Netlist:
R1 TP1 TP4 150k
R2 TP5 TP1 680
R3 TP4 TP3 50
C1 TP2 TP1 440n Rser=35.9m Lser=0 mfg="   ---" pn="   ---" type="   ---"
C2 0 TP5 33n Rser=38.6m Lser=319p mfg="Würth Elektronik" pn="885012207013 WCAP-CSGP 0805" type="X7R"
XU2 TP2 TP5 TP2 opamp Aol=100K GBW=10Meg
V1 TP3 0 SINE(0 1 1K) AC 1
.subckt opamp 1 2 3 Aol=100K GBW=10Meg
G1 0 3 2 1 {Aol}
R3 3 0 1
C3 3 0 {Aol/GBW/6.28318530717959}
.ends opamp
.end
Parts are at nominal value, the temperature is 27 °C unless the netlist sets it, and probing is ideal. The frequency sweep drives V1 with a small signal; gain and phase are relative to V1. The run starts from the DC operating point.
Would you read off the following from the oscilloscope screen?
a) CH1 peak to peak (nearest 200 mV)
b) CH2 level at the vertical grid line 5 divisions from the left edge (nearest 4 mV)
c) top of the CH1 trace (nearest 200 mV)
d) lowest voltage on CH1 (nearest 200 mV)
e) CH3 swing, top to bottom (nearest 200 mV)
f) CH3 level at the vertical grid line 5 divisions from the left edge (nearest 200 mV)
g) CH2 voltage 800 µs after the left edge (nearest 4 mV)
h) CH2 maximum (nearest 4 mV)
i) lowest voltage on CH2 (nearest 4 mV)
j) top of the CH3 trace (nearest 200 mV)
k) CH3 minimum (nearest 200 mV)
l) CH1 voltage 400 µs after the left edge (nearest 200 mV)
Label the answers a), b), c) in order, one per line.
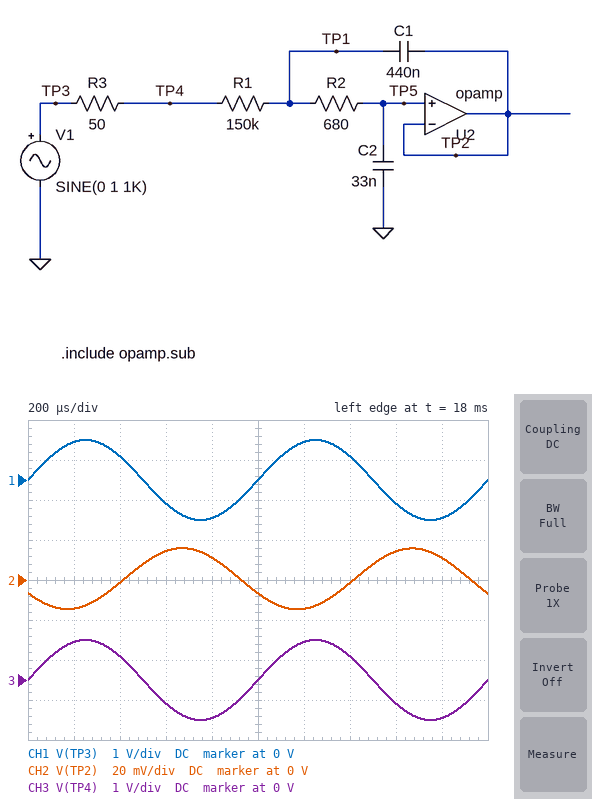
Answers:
a) 2.0 V
b) -8 mV
c) 1.0 V
d) -1.0 V
e) 2.0 V
f) 0 V
g) 12 mV
h) 16 mV
i) -16 mV
j) 1.0 V
k) -1.0 V
l) 600 mV
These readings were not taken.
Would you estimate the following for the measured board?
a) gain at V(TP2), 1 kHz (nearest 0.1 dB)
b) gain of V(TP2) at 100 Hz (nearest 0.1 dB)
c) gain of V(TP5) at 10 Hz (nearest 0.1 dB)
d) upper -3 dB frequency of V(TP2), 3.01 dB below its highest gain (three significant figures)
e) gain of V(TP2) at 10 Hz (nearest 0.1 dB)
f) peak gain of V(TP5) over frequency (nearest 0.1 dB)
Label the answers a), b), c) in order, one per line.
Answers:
a) -36.3 dB
b) -10.0 dB
c) -0.4 dB
d) 34.0 Hz
e) -0.4 dB
f) 0 dB
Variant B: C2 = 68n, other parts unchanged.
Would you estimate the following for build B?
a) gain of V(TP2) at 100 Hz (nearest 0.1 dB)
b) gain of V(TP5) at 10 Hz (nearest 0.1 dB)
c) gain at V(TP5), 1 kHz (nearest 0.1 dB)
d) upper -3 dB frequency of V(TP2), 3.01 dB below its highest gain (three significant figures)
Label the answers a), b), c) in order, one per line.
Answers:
a) -16.2 dB
b) -1.4 dB
c) -42.7 dB
d) 16.0 Hz
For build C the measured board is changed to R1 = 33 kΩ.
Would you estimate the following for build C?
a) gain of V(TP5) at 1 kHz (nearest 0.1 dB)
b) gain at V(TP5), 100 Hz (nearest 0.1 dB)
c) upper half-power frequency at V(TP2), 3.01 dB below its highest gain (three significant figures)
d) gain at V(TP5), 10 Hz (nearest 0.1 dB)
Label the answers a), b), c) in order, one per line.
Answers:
a) -22.8 dB
b) -1.0 dB
c) 186 Hz
d) 0 dB
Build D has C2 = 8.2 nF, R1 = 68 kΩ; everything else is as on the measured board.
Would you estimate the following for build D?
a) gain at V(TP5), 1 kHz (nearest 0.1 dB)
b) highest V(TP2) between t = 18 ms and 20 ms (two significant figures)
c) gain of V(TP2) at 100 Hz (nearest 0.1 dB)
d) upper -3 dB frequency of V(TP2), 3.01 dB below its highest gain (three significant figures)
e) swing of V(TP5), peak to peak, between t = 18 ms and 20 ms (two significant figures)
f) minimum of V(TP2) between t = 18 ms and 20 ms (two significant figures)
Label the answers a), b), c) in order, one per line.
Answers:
a) -16.4 dB
b) 150 mV
c) 0 dB
d) 398 Hz
e) 300 mV
f) -150 mV
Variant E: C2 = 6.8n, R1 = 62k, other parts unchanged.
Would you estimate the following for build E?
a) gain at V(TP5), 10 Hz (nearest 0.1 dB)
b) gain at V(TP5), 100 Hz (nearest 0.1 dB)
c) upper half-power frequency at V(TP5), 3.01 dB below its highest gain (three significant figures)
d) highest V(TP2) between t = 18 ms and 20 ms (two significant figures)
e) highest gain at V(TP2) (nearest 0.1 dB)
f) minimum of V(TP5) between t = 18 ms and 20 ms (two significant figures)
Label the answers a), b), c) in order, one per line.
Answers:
a) 0 dB
b) 0.1 dB
c) 498 Hz
d) 210 mV
e) 0.4 dB
f) -210 mV
